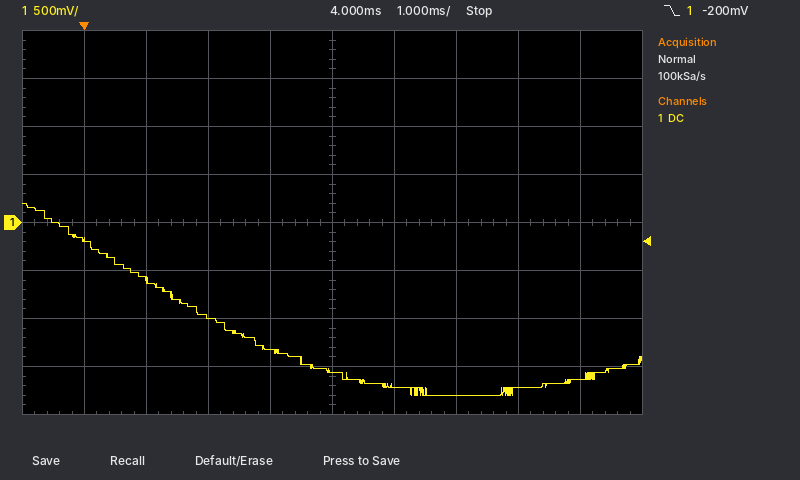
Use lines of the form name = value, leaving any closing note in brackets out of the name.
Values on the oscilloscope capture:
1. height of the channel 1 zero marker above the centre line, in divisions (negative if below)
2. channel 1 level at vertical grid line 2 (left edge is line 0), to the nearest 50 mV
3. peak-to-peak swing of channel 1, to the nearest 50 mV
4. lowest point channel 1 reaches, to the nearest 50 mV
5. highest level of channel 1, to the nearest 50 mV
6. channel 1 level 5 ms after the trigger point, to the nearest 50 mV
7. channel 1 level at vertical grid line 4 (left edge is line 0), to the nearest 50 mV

height of the channel 1 zero marker above the centre line, in divisions = 0.0 div
channel 1 level at vertical grid line 2 (left edge is line 0), to the nearest 50 mV = -600 mV
peak-to-peak swing of channel 1, to the nearest 50 mV = 2.00 V
lowest point channel 1 reaches, to the nearest 50 mV = -1.80 V
highest level of channel 1, to the nearest 50 mV = 200 mV
channel 1 level 5 ms after the trigger point, to the nearest 50 mV = -1.70 V
channel 1 level at vertical grid line 4 (left edge is line 0), to the nearest 50 mV = -1.30 V
